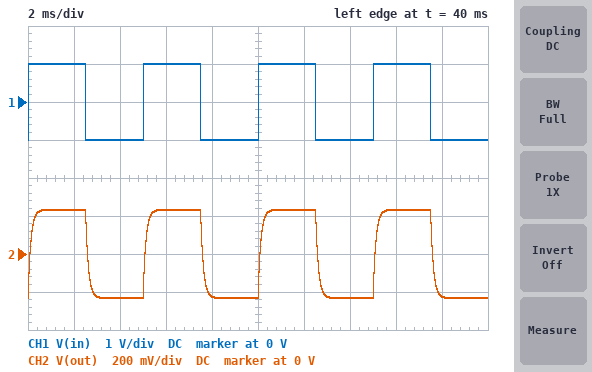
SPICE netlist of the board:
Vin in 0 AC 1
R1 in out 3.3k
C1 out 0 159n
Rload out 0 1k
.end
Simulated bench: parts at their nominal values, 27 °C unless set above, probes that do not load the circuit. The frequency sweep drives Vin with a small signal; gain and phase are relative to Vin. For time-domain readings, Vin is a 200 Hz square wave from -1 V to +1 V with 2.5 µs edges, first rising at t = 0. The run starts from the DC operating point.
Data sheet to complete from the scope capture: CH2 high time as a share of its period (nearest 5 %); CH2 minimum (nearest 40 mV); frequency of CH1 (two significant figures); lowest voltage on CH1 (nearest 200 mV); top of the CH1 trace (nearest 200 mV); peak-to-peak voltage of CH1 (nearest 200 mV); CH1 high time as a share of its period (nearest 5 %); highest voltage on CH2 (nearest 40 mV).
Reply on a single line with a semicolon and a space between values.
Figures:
50 %; -240 mV; 200 Hz; -1.0 V; 1.0 V; 2.0 V; 50 %; 240 mV
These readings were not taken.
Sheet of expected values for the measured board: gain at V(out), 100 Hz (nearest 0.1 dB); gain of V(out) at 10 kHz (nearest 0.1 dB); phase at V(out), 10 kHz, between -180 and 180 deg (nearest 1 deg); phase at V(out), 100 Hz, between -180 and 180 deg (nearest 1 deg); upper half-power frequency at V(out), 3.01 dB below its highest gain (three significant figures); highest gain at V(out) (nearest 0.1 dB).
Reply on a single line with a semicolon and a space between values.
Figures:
-12.7 dB; -30.4 dB; -83 deg; -4 deg; 1.30 kHz; -12.7 dB
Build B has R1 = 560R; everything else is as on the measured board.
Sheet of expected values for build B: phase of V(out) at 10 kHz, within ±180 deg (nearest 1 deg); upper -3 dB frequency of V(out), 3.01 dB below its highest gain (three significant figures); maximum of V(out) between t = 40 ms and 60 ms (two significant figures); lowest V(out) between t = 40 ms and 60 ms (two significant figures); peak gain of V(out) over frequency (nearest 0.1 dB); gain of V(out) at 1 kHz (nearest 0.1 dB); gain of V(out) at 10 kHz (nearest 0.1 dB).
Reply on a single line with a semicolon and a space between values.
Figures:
-74 deg; 2.79 kHz; 640 mV; -640 mV; -3.9 dB; -4.4 dB; -15.3 dB
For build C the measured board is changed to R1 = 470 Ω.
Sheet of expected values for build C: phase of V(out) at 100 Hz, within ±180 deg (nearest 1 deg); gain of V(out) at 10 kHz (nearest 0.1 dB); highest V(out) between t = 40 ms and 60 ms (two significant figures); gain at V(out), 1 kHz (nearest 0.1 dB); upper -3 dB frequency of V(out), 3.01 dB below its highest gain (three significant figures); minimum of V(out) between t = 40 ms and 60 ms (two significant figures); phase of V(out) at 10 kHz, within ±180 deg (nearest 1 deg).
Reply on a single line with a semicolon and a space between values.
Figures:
-2 deg; -13.8 dB; 680 mV; -3.8 dB; 3.13 kHz; -680 mV; -73 deg
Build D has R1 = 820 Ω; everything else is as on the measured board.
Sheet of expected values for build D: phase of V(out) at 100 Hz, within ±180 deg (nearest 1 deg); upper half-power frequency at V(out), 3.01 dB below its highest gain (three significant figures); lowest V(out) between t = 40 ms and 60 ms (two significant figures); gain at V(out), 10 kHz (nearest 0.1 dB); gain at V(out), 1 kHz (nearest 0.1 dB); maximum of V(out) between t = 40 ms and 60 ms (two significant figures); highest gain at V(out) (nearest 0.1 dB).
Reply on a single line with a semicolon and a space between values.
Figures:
-3 deg; 2.22 kHz; -550 mV; -18.5 dB; -6.0 dB; 550 mV; -5.2 dB
